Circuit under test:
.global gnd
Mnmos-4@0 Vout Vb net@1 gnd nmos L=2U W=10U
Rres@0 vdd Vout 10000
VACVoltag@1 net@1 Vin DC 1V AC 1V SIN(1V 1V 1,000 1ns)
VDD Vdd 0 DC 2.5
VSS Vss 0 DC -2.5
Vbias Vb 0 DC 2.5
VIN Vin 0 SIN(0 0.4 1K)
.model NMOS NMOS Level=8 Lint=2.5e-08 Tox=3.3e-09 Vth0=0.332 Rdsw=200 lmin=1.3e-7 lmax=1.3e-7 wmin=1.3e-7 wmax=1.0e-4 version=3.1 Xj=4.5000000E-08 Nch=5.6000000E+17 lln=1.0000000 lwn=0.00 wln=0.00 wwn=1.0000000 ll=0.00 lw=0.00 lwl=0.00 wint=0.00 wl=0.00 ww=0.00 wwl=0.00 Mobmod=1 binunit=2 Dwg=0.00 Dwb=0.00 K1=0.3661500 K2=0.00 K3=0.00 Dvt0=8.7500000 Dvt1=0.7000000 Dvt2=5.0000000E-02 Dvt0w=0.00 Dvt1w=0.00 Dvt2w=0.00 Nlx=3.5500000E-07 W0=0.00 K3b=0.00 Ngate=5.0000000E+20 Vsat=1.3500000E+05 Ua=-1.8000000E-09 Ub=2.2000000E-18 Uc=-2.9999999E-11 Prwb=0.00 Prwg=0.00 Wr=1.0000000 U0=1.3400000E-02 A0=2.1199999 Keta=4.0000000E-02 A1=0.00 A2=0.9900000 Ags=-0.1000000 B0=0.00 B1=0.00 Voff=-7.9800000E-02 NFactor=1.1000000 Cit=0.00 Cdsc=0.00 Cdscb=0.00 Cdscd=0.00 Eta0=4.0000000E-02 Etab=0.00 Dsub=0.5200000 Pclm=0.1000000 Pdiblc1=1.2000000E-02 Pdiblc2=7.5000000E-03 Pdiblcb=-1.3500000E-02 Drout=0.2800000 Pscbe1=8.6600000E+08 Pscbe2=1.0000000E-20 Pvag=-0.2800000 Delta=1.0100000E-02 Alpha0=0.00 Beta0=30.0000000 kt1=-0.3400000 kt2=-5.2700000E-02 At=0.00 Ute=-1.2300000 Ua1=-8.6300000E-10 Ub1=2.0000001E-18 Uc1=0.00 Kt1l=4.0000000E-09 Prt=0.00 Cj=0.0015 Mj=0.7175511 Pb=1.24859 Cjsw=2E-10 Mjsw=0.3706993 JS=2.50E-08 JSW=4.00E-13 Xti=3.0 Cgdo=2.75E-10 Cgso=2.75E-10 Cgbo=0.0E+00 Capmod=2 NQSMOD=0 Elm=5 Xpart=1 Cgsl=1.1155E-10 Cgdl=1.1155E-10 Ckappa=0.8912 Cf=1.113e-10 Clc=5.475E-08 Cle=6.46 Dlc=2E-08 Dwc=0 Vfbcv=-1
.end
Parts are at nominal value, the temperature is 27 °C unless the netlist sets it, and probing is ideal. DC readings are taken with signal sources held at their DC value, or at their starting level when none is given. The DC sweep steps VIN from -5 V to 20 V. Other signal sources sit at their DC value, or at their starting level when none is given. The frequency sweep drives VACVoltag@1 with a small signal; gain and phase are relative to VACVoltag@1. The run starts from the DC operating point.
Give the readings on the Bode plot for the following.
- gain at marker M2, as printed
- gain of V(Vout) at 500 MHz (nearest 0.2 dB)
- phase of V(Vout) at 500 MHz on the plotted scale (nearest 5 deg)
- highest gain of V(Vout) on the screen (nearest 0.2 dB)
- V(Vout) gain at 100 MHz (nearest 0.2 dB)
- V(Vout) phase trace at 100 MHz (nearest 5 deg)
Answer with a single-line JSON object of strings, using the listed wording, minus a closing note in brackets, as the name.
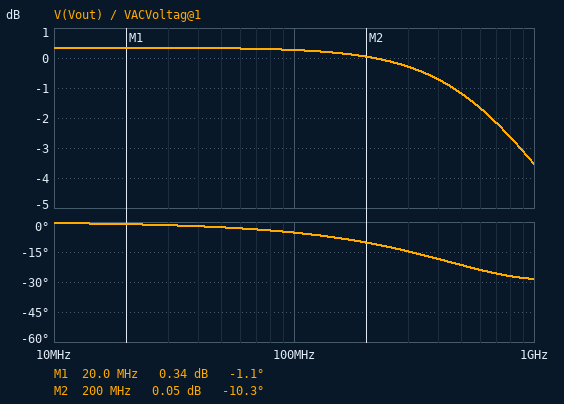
{"gain at marker M2, as printed": "0.05 dB", "gain of V(Vout) at 500 MHz": "-1.2 dB", "phase of V(Vout) at 500 MHz on the plotted scale": "-20 deg", "highest gain of V(Vout) on the screen": "0.4 dB", "V(Vout) gain at 100 MHz": "0.2 dB", "V(Vout) phase trace at 100 MHz": "-5 deg"}
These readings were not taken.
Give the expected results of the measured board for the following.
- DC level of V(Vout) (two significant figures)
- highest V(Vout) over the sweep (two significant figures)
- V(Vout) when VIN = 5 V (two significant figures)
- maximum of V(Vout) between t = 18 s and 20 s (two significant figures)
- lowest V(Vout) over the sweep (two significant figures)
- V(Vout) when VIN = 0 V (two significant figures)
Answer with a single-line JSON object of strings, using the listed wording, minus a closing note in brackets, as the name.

{"DC level of V(Vout)": "1.2 V", "highest V(Vout) over the sweep": "2.5 V", "V(Vout) when VIN = 5 V": "2.5 V", "maximum of V(Vout) between t = 18 s and 20 s": "2.5 V", "lowest V(Vout) over the sweep": "-3.1 V", "V(Vout) when VIN = 0 V": "1.2 V"}
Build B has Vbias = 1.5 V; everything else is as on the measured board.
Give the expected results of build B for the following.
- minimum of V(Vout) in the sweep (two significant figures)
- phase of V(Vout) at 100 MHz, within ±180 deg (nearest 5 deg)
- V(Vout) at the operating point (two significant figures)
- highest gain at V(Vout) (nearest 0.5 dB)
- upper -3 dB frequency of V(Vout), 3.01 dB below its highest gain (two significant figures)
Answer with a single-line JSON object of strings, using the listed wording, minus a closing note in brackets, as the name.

{"minimum of V(Vout) in the sweep": "-3.3 V", "phase of V(Vout) at 100 MHz, within ±180 deg": "0 deg", "V(Vout) at the operating point": "2.5 V", "highest gain at V(Vout)": "-17.5 dB", "upper -3 dB frequency of V(Vout), 3.01 dB below its highest gain": "2.8 GHz"}
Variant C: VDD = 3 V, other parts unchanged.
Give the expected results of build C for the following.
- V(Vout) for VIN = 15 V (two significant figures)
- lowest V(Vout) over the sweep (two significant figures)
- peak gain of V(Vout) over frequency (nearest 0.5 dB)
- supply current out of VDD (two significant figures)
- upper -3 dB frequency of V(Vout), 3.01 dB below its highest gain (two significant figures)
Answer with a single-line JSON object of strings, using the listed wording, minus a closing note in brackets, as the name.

{"V(Vout) for VIN = 15 V": "3.0 V", "lowest V(Vout) over the sweep": "-3.0 V", "peak gain of V(Vout) over frequency": "1.0 dB", "supply current out of VDD": "180 µA", "upper -3 dB frequency of V(Vout), 3.01 dB below its highest gain": "740 MHz"}
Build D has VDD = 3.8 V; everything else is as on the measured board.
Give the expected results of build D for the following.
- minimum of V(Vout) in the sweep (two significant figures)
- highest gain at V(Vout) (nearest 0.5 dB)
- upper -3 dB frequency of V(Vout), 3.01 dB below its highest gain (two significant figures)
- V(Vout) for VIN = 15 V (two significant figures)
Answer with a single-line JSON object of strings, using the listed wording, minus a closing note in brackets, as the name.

{"minimum of V(Vout) in the sweep": "-2.9 V", "highest gain at V(Vout)": "2.5 dB", "upper -3 dB frequency of V(Vout), 3.01 dB below its highest gain": "640 MHz", "V(Vout) for VIN = 15 V": "3.8 V"}
